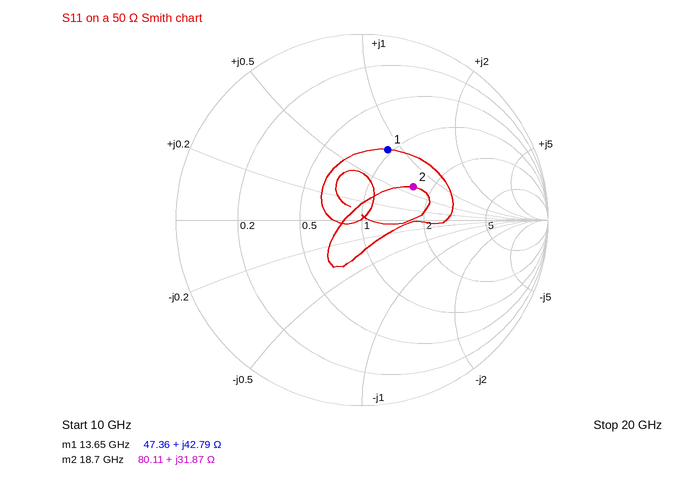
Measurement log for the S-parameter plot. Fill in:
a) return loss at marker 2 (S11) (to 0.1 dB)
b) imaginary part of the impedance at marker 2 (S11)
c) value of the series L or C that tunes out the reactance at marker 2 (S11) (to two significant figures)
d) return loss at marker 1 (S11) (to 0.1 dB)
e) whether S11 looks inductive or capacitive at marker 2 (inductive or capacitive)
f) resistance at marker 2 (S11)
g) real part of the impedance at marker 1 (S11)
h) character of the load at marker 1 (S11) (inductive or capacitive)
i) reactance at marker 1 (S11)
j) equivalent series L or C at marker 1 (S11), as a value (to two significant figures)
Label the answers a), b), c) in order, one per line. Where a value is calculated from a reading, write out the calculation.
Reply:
a) 9.7 dB
b) +31.87 Ω
c) C = 1/(2π × 18.7 GHz × 31.87 Ω) ≈ 267 fF, so 270 fF to two significant figures
d) 7.9 dB
e) inductive
f) 80.11 Ω
g) 47.36 Ω
h) inductive
i) +42.79 Ω
j) L = 42.79 Ω/(2π × 13.65 GHz) ≈ 499 pH, so 500 pH to two significant figures
